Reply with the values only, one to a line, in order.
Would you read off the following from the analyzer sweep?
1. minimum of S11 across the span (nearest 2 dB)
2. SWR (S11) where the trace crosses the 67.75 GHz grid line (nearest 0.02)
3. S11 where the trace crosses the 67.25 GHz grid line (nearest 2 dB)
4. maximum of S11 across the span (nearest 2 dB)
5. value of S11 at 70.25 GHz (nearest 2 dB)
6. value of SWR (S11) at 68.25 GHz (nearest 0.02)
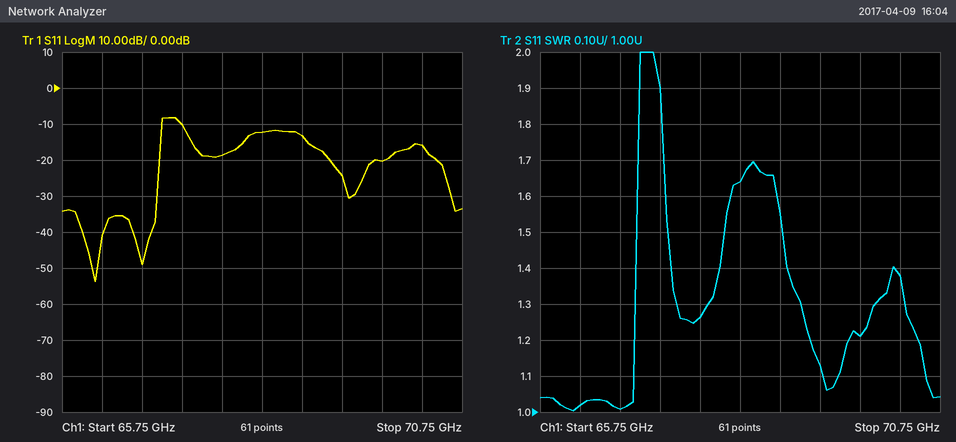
-54 dB
1.26
-10 dB
-8 dB
-16 dB
1.64
